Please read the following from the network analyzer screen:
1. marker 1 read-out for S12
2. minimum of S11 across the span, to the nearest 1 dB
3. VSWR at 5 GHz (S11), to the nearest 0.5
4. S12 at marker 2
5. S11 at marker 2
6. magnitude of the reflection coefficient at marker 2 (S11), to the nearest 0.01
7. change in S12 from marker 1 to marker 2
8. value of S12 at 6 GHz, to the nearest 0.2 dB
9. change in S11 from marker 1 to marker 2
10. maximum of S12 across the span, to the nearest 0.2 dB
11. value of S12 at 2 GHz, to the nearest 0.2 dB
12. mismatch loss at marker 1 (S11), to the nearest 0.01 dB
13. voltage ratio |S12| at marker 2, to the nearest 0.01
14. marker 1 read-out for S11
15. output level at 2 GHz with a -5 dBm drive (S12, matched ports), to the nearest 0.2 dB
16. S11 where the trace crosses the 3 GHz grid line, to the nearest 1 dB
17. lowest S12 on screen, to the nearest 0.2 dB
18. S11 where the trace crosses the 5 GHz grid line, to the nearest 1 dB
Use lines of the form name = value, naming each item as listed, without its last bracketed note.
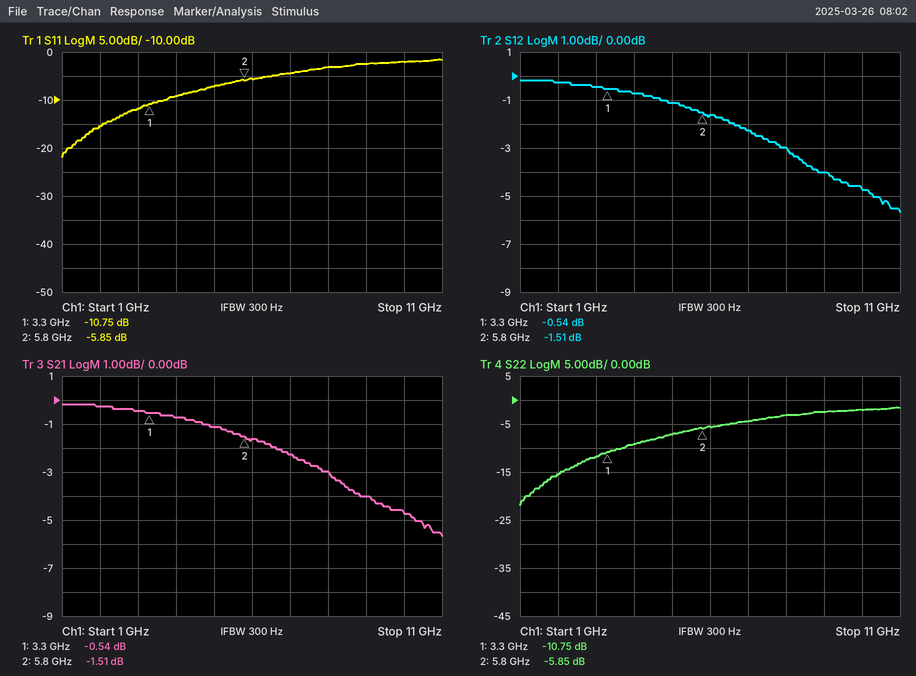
marker 1 read-out for S12 = -0.54 dB
minimum of S11 across the span, to the nearest 1 dB = -22 dB
VSWR at 5 GHz (S11), to the nearest 0.5 = 2.5
S12 at marker 2 = -1.51 dB
S11 at marker 2 = -5.85 dB
magnitude of the reflection coefficient at marker 2 (S11), to the nearest 0.01 = 0.51
change in S12 from marker 1 to marker 2 = -0.97 dB
value of S12 at 6 GHz, to the nearest 0.2 dB = -1.6 dB
change in S11 from marker 1 to marker 2 = 4.90 dB
maximum of S12 across the span, to the nearest 0.2 dB = -0.2 dB
value of S12 at 2 GHz, to the nearest 0.2 dB = -0.2 dB
mismatch loss at marker 1 (S11), to the nearest 0.01 dB = 0.38 dB
voltage ratio |S12| at marker 2, to the nearest 0.01 = 0.84
marker 1 read-out for S11 = -10.75 dB
output level at 2 GHz with a -5 dBm drive (S12, matched ports), to the nearest 0.2 dB = -5.2 dBm
S11 where the trace crosses the 3 GHz grid line, to the nearest 1 dB = -12 dB
lowest S12 on screen, to the nearest 0.2 dB = -5.6 dB
S11 where the trace crosses the 5 GHz grid line, to the nearest 1 dB = -7 dB
